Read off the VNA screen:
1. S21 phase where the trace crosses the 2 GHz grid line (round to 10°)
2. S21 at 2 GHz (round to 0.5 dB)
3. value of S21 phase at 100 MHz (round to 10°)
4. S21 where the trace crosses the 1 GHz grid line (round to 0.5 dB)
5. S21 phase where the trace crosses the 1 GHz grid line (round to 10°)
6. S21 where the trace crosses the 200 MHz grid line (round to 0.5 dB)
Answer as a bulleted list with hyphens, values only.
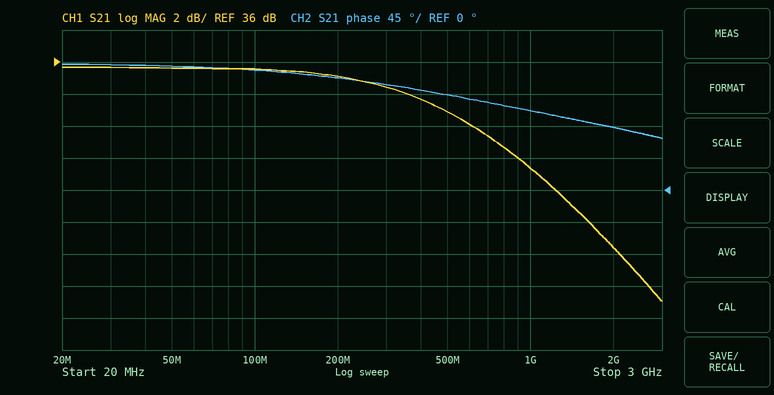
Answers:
- 90°
- 24.5 dB
- 170°
- 29.5 dB
- 110°
- 35.0 dB
